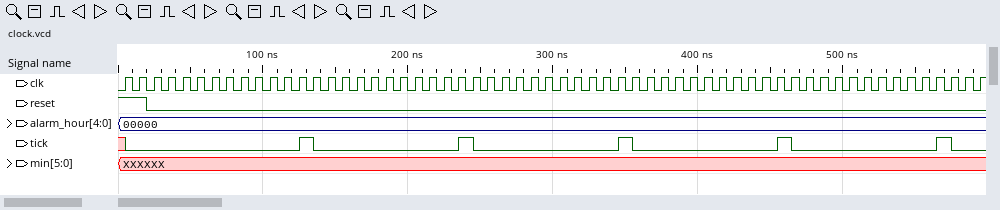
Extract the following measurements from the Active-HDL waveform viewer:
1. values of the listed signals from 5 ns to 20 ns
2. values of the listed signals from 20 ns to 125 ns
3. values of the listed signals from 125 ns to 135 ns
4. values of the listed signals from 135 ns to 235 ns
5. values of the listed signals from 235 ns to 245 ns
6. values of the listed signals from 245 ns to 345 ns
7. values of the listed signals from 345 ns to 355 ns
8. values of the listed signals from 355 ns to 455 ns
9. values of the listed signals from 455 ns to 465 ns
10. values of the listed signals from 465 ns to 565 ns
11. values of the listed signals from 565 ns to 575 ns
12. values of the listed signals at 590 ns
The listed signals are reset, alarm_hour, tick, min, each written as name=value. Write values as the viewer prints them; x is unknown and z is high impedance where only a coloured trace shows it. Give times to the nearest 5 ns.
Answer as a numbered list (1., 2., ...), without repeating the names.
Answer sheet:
1. reset=1, alarm_hour=00000, tick=0, min=XXXXXX
2. reset=0, alarm_hour=00000, tick=0, min=XXXXXX
3. reset=0, alarm_hour=00000, tick=1, min=XXXXXX
4. reset=0, alarm_hour=00000, tick=0, min=XXXXXX
5. reset=0, alarm_hour=00000, tick=1, min=XXXXXX
6. reset=0, alarm_hour=00000, tick=0, min=XXXXXX
7. reset=0, alarm_hour=00000, tick=1, min=XXXXXX
8. reset=0, alarm_hour=00000, tick=0, min=XXXXXX
9. reset=0, alarm_hour=00000, tick=1, min=XXXXXX
10. reset=0, alarm_hour=00000, tick=0, min=XXXXXX
11. reset=0, alarm_hour=00000, tick=1, min=XXXXXX
12. reset=0, alarm_hour=00000, tick=0, min=XXXXXX
